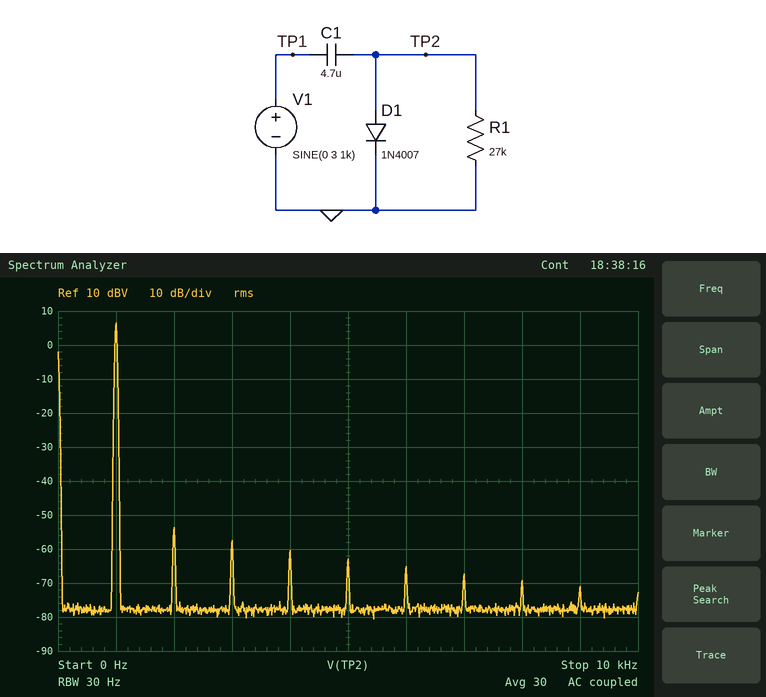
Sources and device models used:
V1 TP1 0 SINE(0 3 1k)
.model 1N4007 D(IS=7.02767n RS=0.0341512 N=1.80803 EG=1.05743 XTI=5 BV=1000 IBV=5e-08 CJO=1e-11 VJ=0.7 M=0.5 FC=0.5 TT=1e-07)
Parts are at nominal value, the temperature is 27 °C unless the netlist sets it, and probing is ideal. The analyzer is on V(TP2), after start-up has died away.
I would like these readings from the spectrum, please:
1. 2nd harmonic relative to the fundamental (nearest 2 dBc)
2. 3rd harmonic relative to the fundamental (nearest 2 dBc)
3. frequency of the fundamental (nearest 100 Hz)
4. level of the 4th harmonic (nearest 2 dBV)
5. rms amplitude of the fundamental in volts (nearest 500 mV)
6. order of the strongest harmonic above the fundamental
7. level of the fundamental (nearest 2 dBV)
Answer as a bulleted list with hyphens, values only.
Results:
- -60 dBc
- -64 dBc
- 1.0 kHz
- -60 dBV
- 2.0 V
- 2
- 6 dBV
